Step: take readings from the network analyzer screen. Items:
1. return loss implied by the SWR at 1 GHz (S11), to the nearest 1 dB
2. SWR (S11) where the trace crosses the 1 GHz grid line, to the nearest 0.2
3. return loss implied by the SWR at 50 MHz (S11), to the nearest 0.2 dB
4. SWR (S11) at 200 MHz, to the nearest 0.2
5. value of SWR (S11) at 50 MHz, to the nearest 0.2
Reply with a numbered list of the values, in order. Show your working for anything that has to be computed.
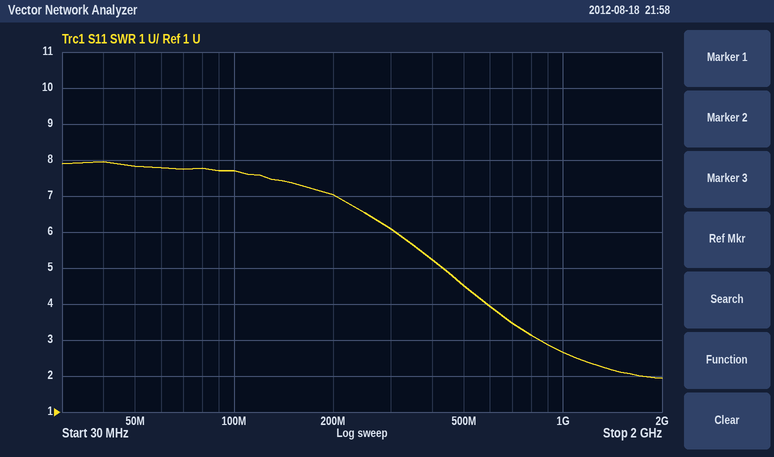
1. −20 log10((2.6 − 1)/(2.6 + 1)) ≈ 7 dB
2. 2.6
3. −20 log10((7.8 − 1)/(7.8 + 1)) ≈ 2.2 dB
4. 7.0
5. 7.8
